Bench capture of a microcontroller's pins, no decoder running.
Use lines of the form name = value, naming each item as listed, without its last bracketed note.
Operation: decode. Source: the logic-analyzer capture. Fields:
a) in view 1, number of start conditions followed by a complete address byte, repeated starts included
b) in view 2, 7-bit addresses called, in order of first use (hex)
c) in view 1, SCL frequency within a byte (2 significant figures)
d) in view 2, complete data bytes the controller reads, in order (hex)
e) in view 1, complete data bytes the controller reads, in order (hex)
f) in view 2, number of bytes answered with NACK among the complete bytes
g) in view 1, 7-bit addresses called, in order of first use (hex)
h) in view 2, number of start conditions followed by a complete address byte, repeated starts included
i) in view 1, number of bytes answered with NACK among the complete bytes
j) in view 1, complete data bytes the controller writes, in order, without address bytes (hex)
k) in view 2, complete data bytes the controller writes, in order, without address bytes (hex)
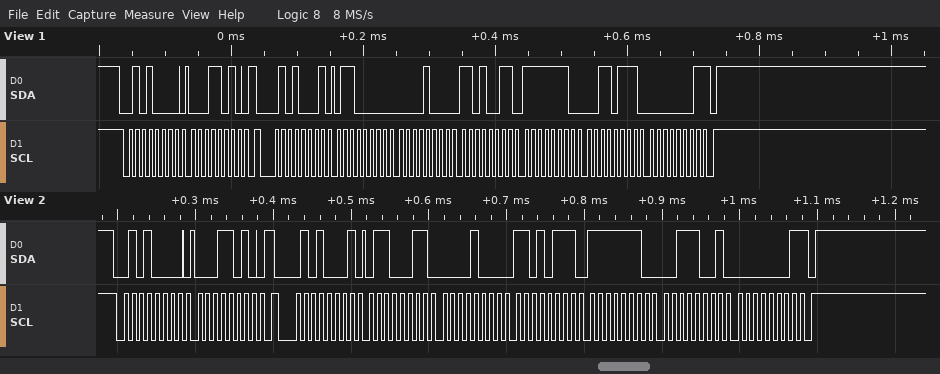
in view 1, number of start conditions followed by a complete address byte, repeated starts included = 2
in view 2, 7-bit addresses called, in order of first use = 0x28
in view 1, SCL frequency within a byte = 100 kHz
in view 2, complete data bytes the controller reads, in order = 63 08 D7 FE 39 01
in view 1, complete data bytes the controller reads, in order = 60 08 D3 FE 37 01
in view 2, number of bytes answered with NACK among the complete bytes = 1
in view 1, 7-bit addresses called, in order of first use = 0x28
in view 2, number of start conditions followed by a complete address byte, repeated starts included = 2
in view 1, number of bytes answered with NACK among the complete bytes = 1
in view 1, complete data bytes the controller writes, in order, without address bytes = 1A
in view 2, complete data bytes the controller writes, in order, without address bytes = 1A
